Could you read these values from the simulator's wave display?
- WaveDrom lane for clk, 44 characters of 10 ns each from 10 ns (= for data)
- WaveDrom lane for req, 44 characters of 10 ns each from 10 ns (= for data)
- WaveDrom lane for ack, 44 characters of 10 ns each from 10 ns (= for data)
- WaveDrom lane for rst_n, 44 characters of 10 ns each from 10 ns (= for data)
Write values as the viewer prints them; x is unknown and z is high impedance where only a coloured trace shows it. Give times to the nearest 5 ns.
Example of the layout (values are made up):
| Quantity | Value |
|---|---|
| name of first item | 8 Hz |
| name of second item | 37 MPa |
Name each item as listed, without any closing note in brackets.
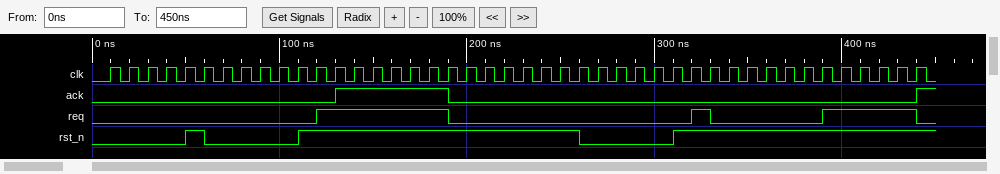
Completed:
| Quantity | Value |
|---|---|
| WaveDrom lane for clk, 44 characters of 10 ns each from 10 ns | {name: 'clk', wave: 'p...........................................'} |
| WaveDrom lane for req, 44 characters of 10 ns each from 10 ns | {name: 'req', wave: '0..........1......0............10.....1....0'} |
| WaveDrom lane for ack, 44 characters of 10 ns each from 10 ns | {name: 'ack', wave: '0...........1.....0........................1'} |
| WaveDrom lane for rst_n, 44 characters of 10 ns each from 10 ns | {name: 'rst_n', wave: '0...10....1..............0....1.............'} |
